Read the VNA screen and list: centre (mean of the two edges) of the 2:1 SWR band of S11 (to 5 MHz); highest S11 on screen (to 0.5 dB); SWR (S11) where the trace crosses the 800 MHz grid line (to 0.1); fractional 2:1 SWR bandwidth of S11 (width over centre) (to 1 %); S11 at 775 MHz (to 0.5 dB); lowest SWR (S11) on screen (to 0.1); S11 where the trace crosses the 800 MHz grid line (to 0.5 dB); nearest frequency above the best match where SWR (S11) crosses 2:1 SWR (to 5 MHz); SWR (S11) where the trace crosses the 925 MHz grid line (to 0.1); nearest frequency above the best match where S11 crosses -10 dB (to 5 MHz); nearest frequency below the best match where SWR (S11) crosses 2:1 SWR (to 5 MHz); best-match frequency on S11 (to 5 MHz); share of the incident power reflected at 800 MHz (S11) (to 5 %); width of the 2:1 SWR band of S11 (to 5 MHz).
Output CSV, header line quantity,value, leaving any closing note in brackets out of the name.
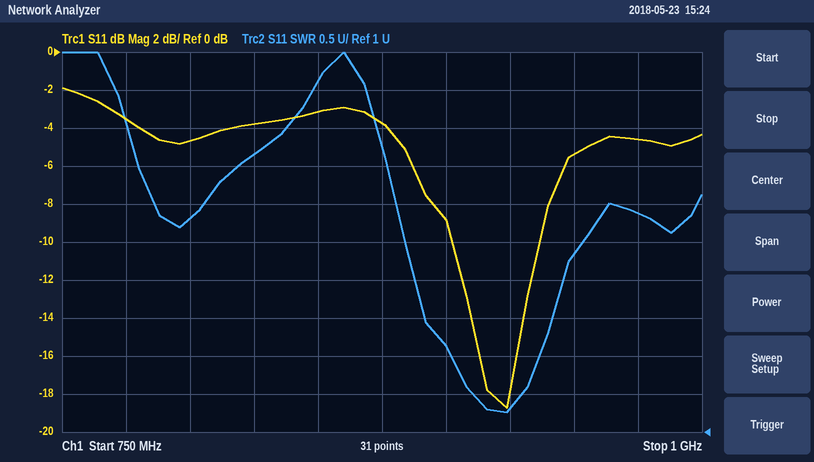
quantity,value
centre (mean of the two edges) of the 2:1 SWR band of S11,920 MHz
highest S11 on screen,-2.0 dB
SWR (S11) where the trace crosses the 800 MHz grid line,3.8
fractional 2:1 SWR bandwidth of S11 (width over centre),4 %
S11 at 775 MHz,-3.5 dB
lowest SWR (S11) on screen,1.3
S11 where the trace crosses the 800 MHz grid line,-4.5 dB
nearest frequency above the best match where SWR (S11) crosses 2:1 SWR,935 MHz
SWR (S11) where the trace crosses the 925 MHz grid line,1.3
nearest frequency above the best match where S11 crosses -10 dB,935 MHz
nearest frequency below the best match where SWR (S11) crosses 2:1 SWR,900 MHz
best-match frequency on S11,925 MHz
share of the incident power reflected at 800 MHz (S11),35 %
width of the 2:1 SWR band of S11,35 MHz
